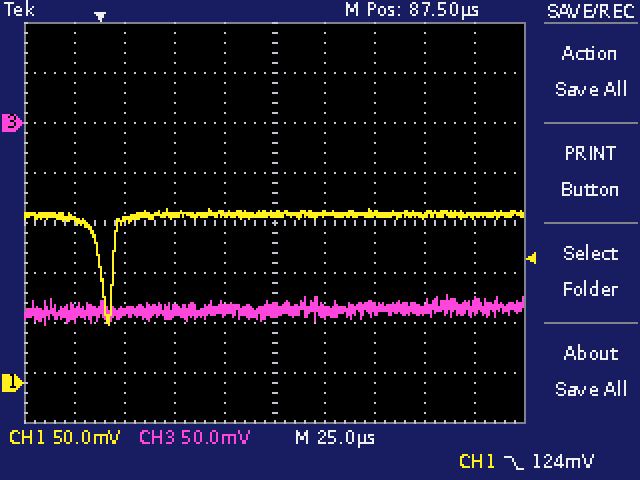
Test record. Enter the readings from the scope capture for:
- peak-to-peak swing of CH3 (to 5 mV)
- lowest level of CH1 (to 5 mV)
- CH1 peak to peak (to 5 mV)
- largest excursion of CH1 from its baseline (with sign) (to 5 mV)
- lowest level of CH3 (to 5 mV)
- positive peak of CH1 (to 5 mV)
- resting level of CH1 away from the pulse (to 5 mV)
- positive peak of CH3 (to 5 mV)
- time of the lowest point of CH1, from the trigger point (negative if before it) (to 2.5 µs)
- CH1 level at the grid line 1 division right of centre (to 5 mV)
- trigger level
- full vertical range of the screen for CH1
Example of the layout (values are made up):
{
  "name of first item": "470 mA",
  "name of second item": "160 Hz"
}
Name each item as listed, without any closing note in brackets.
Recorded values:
{
  "peak-to-peak swing of CH3": "30 mV",
  "lowest level of CH1": "60 mV",
  "CH1 peak to peak": "115 mV",
  "largest excursion of CH1 from its baseline (with sign)": "-110 mV",
  "lowest level of CH3": "-200 mV",
  "positive peak of CH1": "175 mV",
  "resting level of CH1 away from the pulse": "170 mV",
  "positive peak of CH3": "-170 mV",
  "time of the lowest point of CH1, from the trigger point (negative if before it)": "+5.0 µs",
  "CH1 level at the grid line 1 division right of centre": "170 mV",
  "trigger level": "124 mV",
  "full vertical range of the screen for CH1": "400 mV"
}
